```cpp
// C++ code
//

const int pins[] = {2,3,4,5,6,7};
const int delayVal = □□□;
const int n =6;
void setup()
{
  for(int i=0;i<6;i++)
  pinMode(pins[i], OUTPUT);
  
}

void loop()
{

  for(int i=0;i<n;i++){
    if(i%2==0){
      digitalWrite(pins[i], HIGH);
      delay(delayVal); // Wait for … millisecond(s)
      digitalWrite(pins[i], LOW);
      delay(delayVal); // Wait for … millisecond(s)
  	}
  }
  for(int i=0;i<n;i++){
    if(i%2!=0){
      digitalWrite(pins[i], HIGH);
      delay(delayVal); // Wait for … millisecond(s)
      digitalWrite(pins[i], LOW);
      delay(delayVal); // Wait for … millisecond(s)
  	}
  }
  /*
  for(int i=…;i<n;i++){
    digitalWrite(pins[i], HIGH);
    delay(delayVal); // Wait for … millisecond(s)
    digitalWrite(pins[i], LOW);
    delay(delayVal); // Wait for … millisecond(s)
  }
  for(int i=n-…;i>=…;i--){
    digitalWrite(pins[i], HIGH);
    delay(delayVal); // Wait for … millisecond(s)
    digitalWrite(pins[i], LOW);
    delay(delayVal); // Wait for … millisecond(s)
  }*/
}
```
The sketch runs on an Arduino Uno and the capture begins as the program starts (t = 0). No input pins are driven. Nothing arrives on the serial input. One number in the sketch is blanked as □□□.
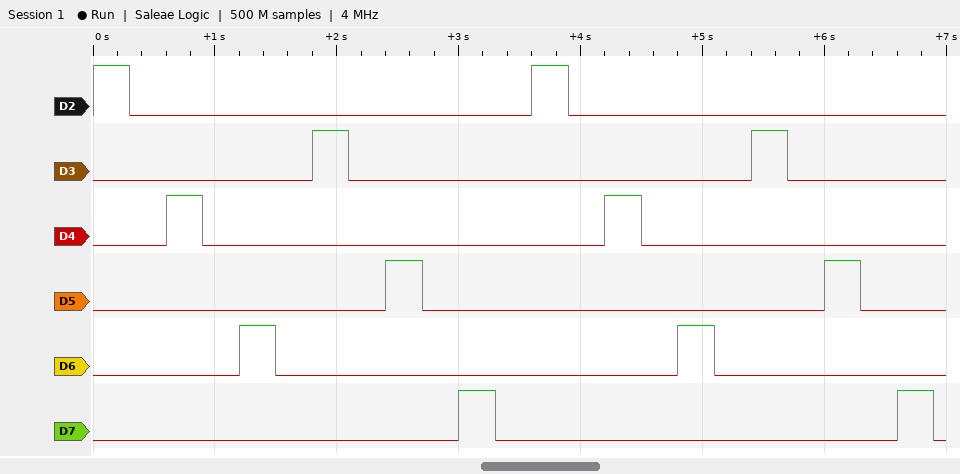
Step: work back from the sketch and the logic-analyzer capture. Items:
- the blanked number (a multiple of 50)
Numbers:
300
